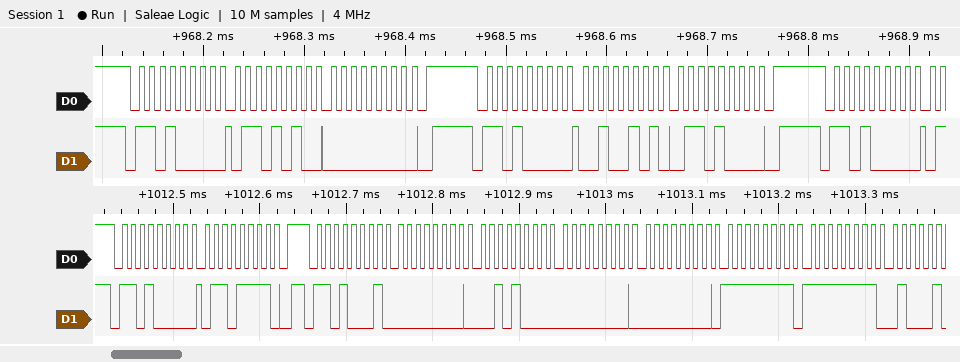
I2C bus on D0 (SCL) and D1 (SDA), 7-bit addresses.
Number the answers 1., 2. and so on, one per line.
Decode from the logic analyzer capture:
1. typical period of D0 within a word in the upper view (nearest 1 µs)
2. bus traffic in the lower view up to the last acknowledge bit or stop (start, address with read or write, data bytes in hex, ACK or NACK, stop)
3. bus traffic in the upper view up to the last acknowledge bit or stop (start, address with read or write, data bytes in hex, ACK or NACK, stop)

1. 10 µs
2. start, address 68 write ACK, 6F ACK, stop, start, address 68 read ACK, 00 ACK, 28 ACK, 00 ACK, 00 ACK, FF ACK, FF ACK
3. start, address 68 write ACK, 6A ACK, 00 ACK, stop, start, address 68 write ACK, 25 ACK, 68 ACK, stop, start, address 68 write ACK
